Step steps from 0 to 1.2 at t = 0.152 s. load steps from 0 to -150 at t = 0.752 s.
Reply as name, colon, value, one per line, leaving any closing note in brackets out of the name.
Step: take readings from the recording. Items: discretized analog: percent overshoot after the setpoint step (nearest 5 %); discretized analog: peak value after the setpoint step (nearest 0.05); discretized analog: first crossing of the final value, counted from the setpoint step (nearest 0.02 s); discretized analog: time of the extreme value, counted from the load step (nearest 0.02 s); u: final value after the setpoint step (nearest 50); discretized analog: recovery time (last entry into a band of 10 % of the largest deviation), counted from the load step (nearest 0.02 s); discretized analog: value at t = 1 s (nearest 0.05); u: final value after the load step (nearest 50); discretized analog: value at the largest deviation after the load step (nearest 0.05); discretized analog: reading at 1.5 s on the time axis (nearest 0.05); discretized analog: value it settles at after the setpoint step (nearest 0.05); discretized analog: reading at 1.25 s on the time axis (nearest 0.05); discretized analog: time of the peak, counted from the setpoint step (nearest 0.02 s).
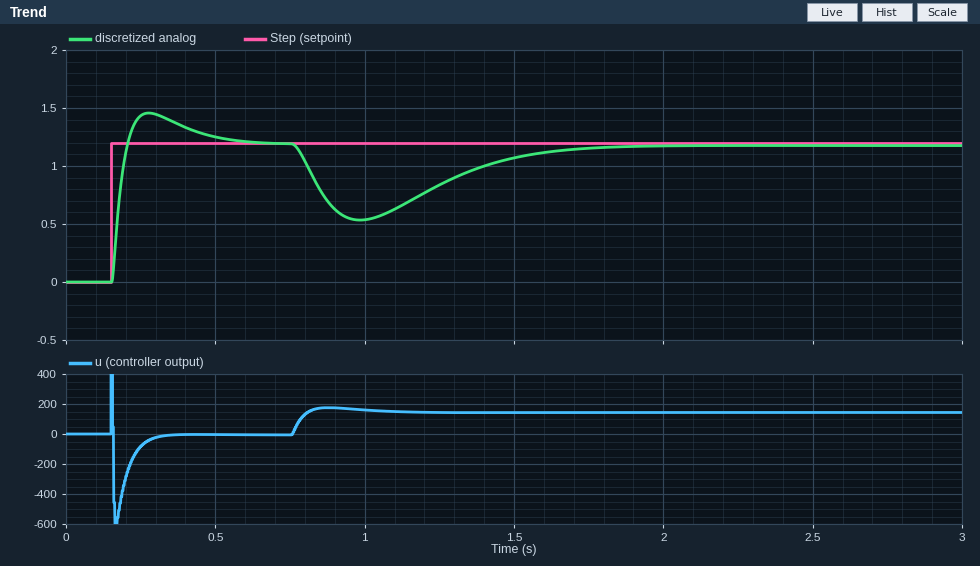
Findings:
discretized analog: percent overshoot after the setpoint step: 20 %
discretized analog: peak value after the setpoint step: 1.45
discretized analog: first crossing of the final value, counted from the setpoint step: 0.06 s
discretized analog: time of the extreme value, counted from the load step: 0.24 s
u: final value after the setpoint step: 0
discretized analog: recovery time (last entry into a band of 10 % of the largest deviation), counted from the load step: 0.84 s
discretized analog: value at t = 1 s: 0.55
u: final value after the load step: 150
discretized analog: value at the largest deviation after the load step: 0.55
discretized analog: reading at 1.5 s on the time axis: 1.05
discretized analog: value it settles at after the setpoint step: 1.20
discretized analog: reading at 1.25 s on the time axis: 0.85
discretized analog: time of the peak, counted from the setpoint step: 0.12 s
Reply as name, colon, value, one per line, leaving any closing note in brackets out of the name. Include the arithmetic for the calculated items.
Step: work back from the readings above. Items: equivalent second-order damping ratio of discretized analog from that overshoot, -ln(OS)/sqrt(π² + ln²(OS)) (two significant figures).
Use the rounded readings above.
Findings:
equivalent second-order damping ratio of discretized analog from that overshoot, -ln(OS)/sqrt(π² + ln²(OS)): ln(0.2) = -1.609; 1.609 / sqrt(9.870 + 2.590) = 0.46
